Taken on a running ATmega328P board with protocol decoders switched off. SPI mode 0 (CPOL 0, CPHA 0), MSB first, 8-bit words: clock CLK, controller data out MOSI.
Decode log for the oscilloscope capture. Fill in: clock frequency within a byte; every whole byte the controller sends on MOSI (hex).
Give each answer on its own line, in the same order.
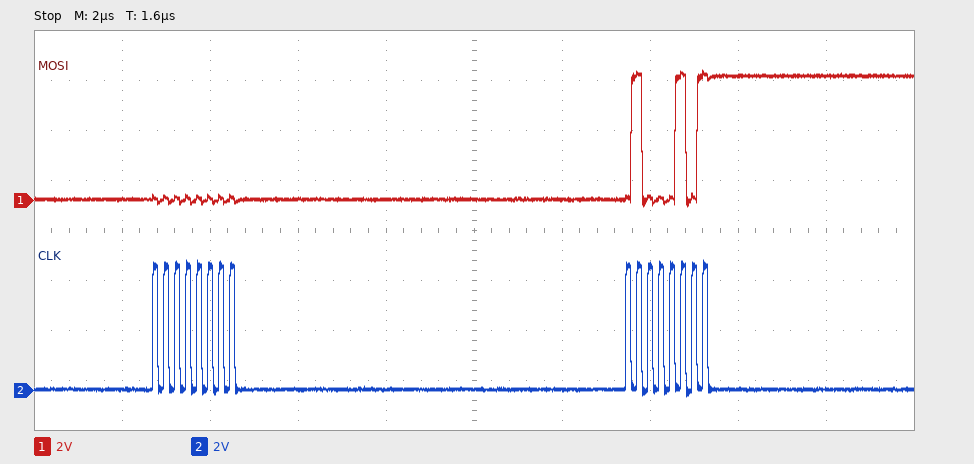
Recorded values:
4 MHz
00 45
